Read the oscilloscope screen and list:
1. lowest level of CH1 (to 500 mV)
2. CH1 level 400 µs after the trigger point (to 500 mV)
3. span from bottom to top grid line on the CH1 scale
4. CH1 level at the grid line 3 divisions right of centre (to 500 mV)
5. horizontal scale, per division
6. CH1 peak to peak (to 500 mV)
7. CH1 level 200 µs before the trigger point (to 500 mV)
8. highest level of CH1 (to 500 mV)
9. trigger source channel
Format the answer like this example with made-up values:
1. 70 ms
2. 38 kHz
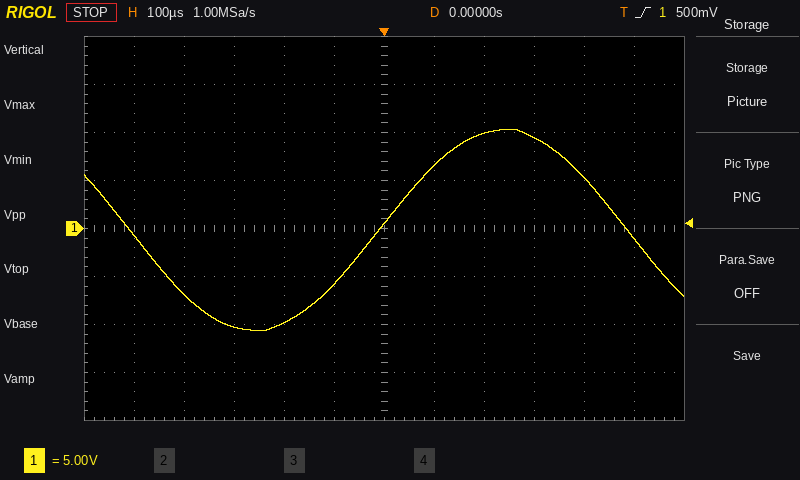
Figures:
1. -10.5 V
2. 5.5 V
3. 40 V
4. 9.5 V
5. 100 µs
6. 21.0 V
7. -10.0 V
8. 10.5 V
9. CH1
